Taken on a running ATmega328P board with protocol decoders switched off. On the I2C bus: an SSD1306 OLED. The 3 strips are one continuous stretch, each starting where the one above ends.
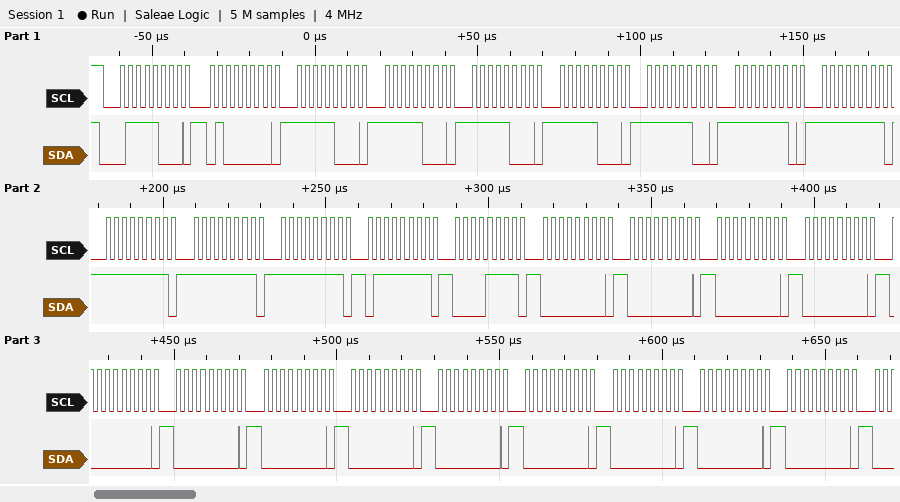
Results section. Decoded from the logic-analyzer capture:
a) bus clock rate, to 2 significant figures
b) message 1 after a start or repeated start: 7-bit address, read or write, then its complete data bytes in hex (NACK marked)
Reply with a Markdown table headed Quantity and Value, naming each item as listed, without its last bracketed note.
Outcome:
| Quantity | Value |
|---|---|
| bus clock rate, to 2 significant figures | 400 kHz |
| message 1 after a start or repeated start: 7-bit address, read or write, then its complete data bytes in hex | 0x3C write: 40 F8 F8 F8 F8 FC FE FF FF FF FF 7F 0F 00 00 00 00 00 00 00 00 00 00 00 00 00 |
